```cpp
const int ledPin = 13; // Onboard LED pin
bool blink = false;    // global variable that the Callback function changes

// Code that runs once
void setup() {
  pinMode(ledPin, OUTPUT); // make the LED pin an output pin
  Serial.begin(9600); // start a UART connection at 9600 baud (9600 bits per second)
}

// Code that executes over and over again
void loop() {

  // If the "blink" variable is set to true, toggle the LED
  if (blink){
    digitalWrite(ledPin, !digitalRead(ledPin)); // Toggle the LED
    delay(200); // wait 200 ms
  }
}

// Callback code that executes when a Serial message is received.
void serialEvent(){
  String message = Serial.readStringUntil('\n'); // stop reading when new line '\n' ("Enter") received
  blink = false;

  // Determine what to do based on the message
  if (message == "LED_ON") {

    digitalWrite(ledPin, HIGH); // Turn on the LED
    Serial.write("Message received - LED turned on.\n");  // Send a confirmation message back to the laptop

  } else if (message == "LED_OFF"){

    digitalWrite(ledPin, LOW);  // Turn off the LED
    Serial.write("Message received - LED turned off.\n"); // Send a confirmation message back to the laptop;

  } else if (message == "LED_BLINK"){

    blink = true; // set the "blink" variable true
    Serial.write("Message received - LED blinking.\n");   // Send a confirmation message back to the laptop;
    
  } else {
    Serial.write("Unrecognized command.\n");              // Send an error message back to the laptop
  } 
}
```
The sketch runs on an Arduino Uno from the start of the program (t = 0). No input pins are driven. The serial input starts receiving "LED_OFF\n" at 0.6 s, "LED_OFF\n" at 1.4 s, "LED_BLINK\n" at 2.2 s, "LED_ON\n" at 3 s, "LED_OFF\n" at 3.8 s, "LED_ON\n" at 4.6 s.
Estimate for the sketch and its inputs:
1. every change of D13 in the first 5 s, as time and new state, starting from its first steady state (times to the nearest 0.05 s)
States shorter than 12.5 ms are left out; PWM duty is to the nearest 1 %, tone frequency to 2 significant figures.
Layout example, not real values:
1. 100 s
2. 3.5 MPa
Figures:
1. 0 s low; 2.2 s high; 2.4 s low; 2.6 s high; 2.8 s low; 3 s high; 3.8 s low; 4.6 s high
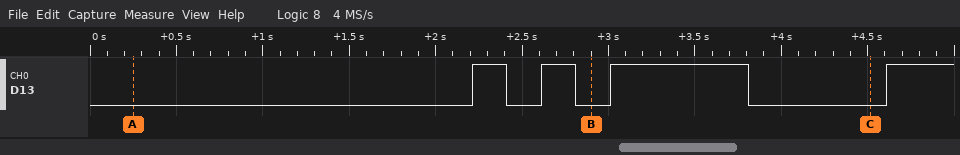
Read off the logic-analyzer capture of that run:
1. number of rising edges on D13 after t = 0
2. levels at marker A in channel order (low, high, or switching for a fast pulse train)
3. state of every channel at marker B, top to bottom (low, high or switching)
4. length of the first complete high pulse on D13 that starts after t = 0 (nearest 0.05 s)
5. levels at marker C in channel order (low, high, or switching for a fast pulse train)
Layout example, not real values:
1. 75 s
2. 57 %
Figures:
1. 4
2. D13 low
3. D13 low
4. 0.20 s
5. D13 low
